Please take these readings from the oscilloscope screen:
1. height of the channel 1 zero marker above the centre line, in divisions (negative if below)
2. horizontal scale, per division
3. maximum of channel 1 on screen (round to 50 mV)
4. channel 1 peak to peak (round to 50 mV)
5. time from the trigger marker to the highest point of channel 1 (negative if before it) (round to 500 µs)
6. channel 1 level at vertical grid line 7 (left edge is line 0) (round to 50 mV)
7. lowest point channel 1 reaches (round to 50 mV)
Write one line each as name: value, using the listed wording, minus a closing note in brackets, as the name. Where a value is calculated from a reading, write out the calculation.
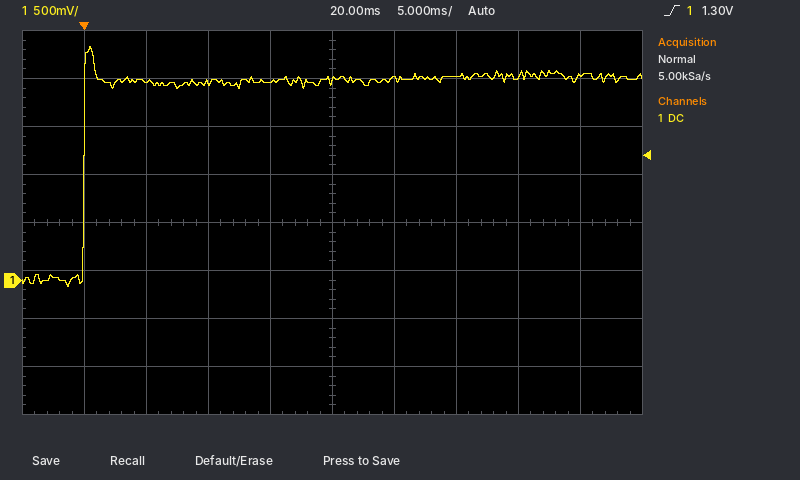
height of the channel 1 zero marker above the centre line, in divisions: -1.2 div
horizontal scale, per division: 5 ms
maximum of channel 1 on screen: 2.45 V
channel 1 peak to peak: 2.45 V − (-50 mV) = 2.50 V
time from the trigger marker to the highest point of channel 1 (negative if before it): +500 µs
channel 1 level at vertical grid line 7 (left edge is line 0): 2.10 V
lowest point channel 1 reaches: -50 mV
